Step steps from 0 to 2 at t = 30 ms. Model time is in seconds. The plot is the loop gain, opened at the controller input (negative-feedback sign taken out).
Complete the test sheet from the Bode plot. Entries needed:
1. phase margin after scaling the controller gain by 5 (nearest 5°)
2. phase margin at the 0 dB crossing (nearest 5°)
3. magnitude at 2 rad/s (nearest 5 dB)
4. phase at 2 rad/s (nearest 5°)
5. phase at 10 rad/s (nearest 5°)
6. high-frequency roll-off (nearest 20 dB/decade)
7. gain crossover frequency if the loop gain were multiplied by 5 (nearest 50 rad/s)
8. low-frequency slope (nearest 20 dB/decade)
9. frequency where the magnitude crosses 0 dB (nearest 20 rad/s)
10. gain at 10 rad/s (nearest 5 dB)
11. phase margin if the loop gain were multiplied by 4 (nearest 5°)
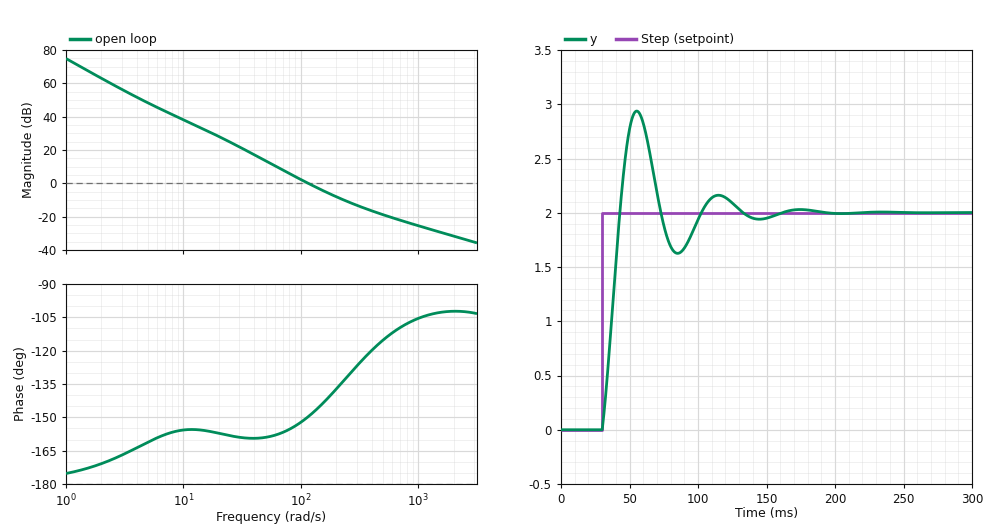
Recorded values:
55°
30°
65 dB
-170°
-155°
-20 dB/decade
300 rad/s
-40 dB/decade
120 rad/s
40 dB
50°
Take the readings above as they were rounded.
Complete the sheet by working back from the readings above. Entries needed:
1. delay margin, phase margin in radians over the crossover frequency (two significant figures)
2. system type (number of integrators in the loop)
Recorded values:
0.0044 s
2
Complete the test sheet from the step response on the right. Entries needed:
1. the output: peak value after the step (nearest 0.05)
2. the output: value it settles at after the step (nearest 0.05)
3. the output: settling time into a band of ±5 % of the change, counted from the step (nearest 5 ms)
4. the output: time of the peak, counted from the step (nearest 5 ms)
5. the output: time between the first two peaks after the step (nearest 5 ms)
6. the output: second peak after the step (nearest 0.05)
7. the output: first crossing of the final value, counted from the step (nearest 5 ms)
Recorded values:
2.95
2.00
95 ms
25 ms
60 ms
2.15
15 ms
